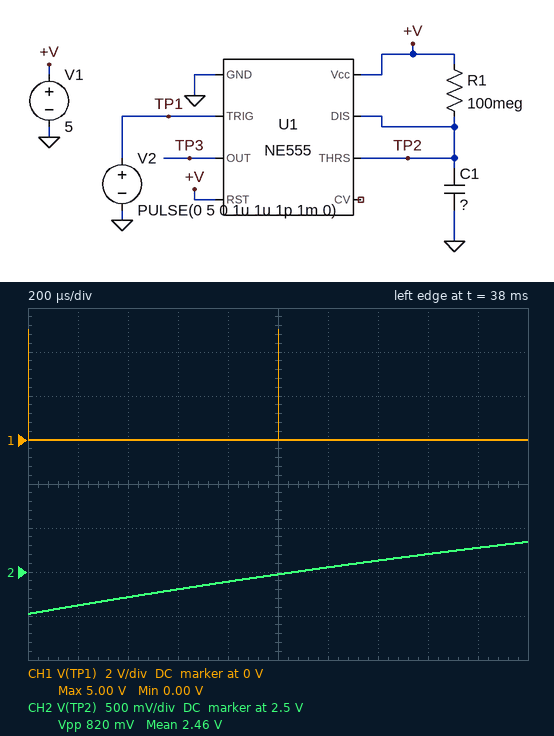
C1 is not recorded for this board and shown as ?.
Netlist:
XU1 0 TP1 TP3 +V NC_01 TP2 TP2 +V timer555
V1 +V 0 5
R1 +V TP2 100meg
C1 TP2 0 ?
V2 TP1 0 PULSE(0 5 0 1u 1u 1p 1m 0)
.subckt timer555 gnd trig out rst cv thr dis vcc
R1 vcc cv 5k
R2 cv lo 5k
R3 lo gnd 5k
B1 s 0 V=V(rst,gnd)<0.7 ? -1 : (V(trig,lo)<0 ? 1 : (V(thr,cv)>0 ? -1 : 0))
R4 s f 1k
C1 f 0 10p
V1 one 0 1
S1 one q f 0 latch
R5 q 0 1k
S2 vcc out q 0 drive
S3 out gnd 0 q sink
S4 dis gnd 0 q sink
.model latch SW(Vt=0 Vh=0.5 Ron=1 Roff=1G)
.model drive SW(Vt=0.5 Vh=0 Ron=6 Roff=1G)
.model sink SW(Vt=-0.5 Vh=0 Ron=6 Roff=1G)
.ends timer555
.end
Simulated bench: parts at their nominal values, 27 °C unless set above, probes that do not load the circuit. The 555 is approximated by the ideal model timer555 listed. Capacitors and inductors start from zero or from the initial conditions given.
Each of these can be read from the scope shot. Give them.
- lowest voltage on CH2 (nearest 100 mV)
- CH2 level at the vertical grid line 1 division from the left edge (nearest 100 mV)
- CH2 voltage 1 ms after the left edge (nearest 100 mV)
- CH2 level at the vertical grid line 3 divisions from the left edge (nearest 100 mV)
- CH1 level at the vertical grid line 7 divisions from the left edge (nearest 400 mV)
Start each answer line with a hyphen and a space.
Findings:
- 2.0 V
- 2.1 V
- 2.5 V
- 2.3 V
- 0 V
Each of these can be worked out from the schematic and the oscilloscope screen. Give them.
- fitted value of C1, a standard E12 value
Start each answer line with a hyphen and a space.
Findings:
- 56 pF
